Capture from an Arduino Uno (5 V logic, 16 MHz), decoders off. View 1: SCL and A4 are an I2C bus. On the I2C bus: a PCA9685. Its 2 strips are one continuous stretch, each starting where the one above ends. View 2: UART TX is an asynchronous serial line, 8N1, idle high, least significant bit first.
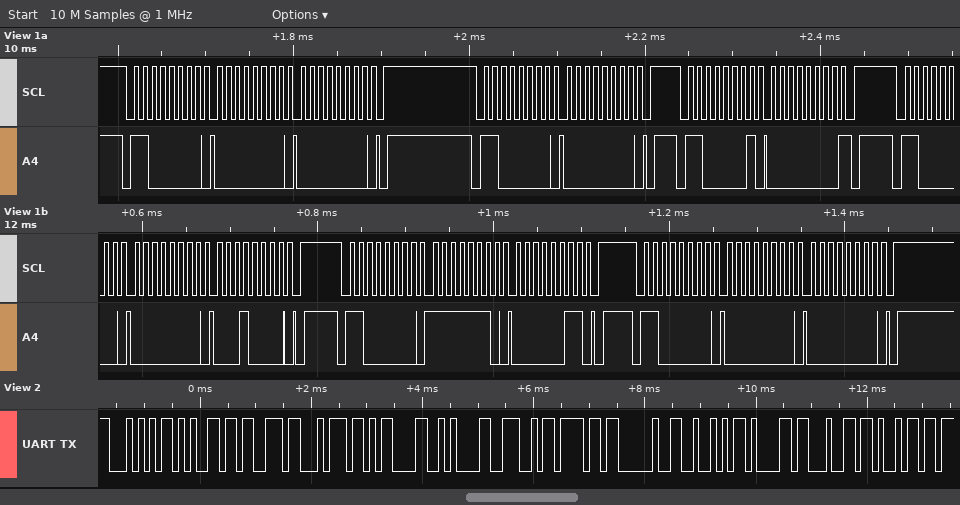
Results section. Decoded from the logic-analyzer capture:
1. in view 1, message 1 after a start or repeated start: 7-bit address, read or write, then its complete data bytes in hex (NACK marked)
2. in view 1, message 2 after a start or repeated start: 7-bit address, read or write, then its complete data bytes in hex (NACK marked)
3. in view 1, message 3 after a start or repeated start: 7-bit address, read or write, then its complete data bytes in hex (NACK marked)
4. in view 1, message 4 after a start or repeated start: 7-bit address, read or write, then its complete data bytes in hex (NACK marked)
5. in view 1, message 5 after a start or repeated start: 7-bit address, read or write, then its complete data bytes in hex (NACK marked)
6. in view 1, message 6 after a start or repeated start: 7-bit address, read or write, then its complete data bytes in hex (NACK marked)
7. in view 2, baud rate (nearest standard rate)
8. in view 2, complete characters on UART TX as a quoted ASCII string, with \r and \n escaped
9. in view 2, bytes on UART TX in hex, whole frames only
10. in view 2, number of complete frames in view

0x60 write: 00 00
0x60 write: 00
0x60 read: 00 NACK
0x60 write: 00 10
0x60 write: FE 03
0x60 write: 00 00
9600 baud
"Test\r\nNo Radi"
54 65 73 74 0D 0A 4E 6F 20 52 61 64 69
13
